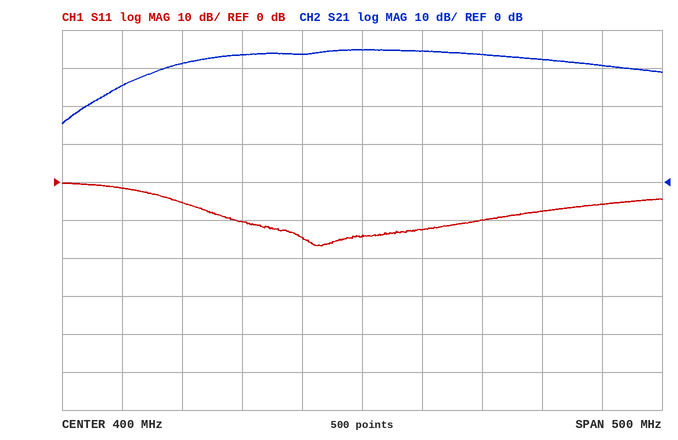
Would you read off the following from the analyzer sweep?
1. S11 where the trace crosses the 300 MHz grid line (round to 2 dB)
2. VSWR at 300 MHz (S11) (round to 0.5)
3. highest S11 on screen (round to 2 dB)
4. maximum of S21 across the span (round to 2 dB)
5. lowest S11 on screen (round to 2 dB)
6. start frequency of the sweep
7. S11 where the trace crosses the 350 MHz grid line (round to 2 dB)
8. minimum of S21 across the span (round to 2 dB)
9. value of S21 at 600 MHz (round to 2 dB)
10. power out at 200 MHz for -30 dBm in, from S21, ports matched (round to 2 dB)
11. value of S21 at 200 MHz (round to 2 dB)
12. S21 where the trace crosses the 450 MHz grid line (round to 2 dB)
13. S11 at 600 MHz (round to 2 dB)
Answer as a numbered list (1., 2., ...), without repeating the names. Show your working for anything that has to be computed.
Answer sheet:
1. -10 dB
2. |Γ| = 10^(-10/20) = 0.3162; VSWR = (1 + 0.3162)/(1 − 0.3162) ≈ 1.92, so 2.0 to the nearest 0.5
3. 0 dB
4. 34 dB
5. -16 dB
6. 150 MHz
7. -14 dB
8. 16 dB
9. 30 dB
10. -30 dBm + (26 dB) = -4 dBm
11. 26 dB
12. 34 dB
13. -6 dB
